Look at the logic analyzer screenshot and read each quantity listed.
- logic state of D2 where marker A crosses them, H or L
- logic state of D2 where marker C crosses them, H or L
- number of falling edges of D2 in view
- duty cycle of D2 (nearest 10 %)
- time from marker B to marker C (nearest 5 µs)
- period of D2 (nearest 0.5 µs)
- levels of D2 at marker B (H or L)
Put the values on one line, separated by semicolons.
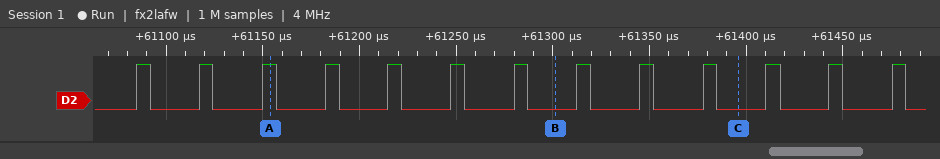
D2=H; D2=L; 13; 20 %; 95 µs; 32.5 µs; D2=L
